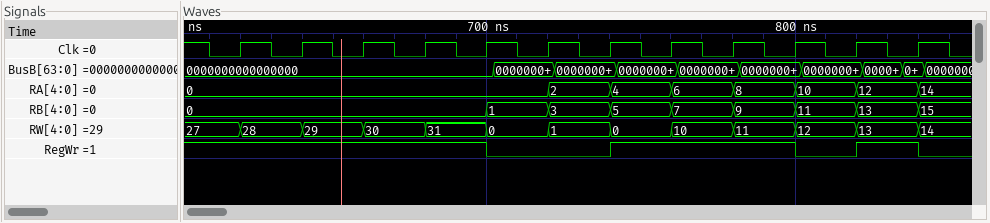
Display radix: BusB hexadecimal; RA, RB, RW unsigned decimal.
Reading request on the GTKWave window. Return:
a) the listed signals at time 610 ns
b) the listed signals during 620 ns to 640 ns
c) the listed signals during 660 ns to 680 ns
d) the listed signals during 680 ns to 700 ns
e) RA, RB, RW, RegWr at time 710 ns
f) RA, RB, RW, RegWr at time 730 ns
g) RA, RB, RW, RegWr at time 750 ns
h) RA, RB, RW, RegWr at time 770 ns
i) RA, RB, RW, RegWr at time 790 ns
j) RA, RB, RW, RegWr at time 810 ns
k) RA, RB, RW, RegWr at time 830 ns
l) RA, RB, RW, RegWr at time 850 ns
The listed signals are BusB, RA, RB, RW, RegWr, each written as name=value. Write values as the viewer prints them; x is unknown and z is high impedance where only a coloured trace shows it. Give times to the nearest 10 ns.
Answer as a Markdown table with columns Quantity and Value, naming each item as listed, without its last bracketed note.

| Quantity | Value |
|---|---|
| the listed signals at time 610 ns | BusB=0000000000000000, RA=0, RB=0, RW=27, RegWr=1 |
| the listed signals during 620 ns to 640 ns | BusB=0000000000000000, RA=0, RB=0, RW=28, RegWr=1 |
| the listed signals during 660 ns to 680 ns | BusB=0000000000000000, RA=0, RB=0, RW=30, RegWr=1 |
| the listed signals during 680 ns to 700 ns | BusB=0000000000000000, RA=0, RB=0, RW=31, RegWr=1 |
| RA, RB, RW, RegWr at time 710 ns | RA=0, RB=1, RW=0, RegWr=0 |
| RA, RB, RW, RegWr at time 730 ns | RA=2, RB=3, RW=1, RegWr=0 |
| RA, RB, RW, RegWr at time 750 ns | RA=4, RB=5, RW=0, RegWr=1 |
| RA, RB, RW, RegWr at time 770 ns | RA=6, RB=7, RW=10, RegWr=1 |
| RA, RB, RW, RegWr at time 790 ns | RA=8, RB=9, RW=11, RegWr=1 |
| RA, RB, RW, RegWr at time 810 ns | RA=10, RB=11, RW=12, RegWr=0 |
| RA, RB, RW, RegWr at time 830 ns | RA=12, RB=13, RW=13, RegWr=1 |
| RA, RB, RW, RegWr at time 850 ns | RA=14, RB=15, RW=14, RegWr=0 |
